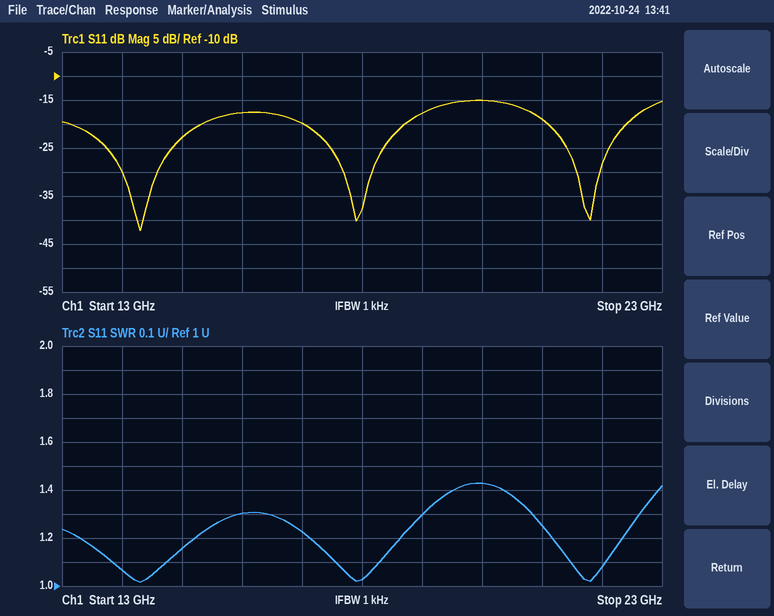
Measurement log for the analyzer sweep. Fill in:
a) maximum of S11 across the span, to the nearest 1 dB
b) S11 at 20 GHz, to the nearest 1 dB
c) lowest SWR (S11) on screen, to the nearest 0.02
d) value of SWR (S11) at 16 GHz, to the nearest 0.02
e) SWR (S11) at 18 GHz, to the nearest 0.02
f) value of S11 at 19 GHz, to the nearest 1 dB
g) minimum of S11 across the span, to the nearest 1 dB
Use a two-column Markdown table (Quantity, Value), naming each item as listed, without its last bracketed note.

| Quantity | Value |
|---|---|
| maximum of S11 across the span, to the nearest 1 dB | -15 dB |
| S11 at 20 GHz, to the nearest 1 dB | -15 dB |
| lowest SWR (S11) on screen, to the nearest 0.02 | 1.02 |
| value of SWR (S11) at 16 GHz, to the nearest 0.02 | 1.30 |
| SWR (S11) at 18 GHz, to the nearest 0.02 | 1.02 |
| value of S11 at 19 GHz, to the nearest 1 dB | -18 dB |
| minimum of S11 across the span, to the nearest 1 dB | -42 dB |
